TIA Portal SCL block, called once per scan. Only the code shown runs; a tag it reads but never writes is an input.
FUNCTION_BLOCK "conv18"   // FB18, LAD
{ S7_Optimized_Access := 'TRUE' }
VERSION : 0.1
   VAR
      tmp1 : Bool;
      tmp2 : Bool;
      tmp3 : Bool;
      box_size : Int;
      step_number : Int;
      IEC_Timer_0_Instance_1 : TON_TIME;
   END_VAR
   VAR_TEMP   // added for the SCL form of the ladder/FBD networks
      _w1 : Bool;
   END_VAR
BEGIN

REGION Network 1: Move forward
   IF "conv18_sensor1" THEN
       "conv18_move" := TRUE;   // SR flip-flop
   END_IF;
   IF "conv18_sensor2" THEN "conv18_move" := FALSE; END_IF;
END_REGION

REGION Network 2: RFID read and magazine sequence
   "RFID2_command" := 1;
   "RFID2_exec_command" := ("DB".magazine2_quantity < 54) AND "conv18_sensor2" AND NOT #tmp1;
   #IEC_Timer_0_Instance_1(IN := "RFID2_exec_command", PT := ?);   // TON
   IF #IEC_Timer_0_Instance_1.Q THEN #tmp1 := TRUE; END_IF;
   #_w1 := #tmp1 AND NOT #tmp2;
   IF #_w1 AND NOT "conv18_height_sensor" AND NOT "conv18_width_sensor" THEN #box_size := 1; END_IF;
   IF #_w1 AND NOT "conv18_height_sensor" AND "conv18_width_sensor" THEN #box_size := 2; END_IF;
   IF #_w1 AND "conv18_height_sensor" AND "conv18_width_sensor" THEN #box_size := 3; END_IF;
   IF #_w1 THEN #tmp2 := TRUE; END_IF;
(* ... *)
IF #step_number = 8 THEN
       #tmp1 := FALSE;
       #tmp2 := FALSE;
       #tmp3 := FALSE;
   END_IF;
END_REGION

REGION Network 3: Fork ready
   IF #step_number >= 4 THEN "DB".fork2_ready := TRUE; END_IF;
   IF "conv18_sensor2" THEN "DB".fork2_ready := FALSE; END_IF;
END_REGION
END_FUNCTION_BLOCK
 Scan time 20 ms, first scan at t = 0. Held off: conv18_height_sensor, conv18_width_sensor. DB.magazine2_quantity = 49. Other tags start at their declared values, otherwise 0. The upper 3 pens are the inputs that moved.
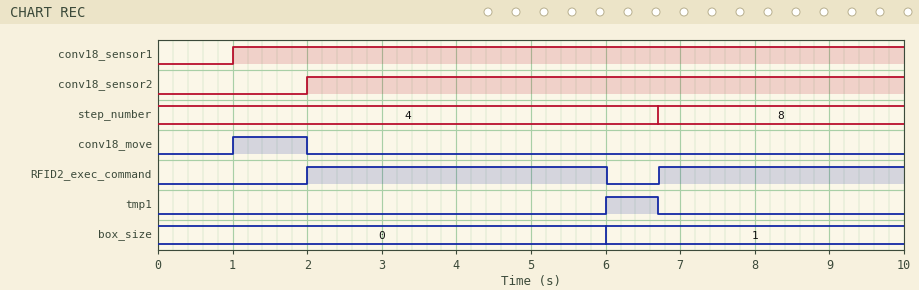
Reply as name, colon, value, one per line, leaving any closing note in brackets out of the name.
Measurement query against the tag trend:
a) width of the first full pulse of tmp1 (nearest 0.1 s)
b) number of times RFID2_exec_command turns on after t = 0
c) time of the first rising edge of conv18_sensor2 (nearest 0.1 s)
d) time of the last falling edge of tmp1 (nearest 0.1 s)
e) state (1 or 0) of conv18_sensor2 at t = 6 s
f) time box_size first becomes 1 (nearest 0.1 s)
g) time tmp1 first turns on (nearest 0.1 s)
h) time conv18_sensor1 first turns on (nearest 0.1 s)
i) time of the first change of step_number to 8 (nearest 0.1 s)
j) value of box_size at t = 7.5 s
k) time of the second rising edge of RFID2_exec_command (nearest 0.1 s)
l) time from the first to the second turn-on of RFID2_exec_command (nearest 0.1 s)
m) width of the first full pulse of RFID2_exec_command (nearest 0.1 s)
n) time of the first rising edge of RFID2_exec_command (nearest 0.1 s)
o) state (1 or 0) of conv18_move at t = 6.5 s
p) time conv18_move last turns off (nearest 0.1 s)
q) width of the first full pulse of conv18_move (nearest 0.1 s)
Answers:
width of the first full pulse of tmp1: 0.7 s
number of times RFID2_exec_command turns on after t = 0: 2
time of the first rising edge of conv18_sensor2: 2.0 s
time of the last falling edge of tmp1: 6.7 s
state (1 or 0) of conv18_sensor2 at t = 6 s: 1
time box_size first becomes 1: 6.0 s
time tmp1 first turns on: 6.0 s
time conv18_sensor1 first turns on: 1.0 s
time of the first change of step_number to 8: 6.7 s
value of box_size at t = 7.5 s: 1
time of the second rising edge of RFID2_exec_command: 6.7 s
time from the first to the second turn-on of RFID2_exec_command: 4.7 s
width of the first full pulse of RFID2_exec_command: 4.0 s
time of the first rising edge of RFID2_exec_command: 2.0 s
state (1 or 0) of conv18_move at t = 6.5 s: 0
time conv18_move last turns off: 2.0 s
width of the first full pulse of conv18_move: 1.0 s
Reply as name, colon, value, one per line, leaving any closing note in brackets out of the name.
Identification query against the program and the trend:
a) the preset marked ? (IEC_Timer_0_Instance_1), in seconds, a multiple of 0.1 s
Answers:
the preset marked ? (IEC_Timer_0_Instance_1), in seconds, a multiple of 0.1 s: 4.0 s
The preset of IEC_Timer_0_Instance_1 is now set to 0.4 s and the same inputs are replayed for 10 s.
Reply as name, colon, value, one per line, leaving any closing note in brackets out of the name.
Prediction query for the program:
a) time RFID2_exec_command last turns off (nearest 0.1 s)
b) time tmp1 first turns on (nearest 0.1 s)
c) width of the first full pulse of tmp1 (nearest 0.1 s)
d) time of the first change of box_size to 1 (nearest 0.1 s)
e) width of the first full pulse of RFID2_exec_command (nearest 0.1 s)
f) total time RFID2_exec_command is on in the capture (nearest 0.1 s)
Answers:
time RFID2_exec_command last turns off: 2.4 s
time tmp1 first turns on: 2.4 s
width of the first full pulse of tmp1: 4.3 s
time of the first change of box_size to 1: 2.4 s
width of the first full pulse of RFID2_exec_command: 0.4 s
total time RFID2_exec_command is on in the capture: 3.7 s
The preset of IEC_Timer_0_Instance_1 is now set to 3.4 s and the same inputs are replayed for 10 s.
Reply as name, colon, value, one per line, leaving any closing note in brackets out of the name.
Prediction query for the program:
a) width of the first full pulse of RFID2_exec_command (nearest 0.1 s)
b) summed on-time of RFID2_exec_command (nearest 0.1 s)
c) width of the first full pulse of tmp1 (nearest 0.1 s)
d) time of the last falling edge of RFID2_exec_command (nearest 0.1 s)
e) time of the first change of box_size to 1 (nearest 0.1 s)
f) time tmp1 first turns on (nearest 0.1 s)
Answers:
width of the first full pulse of RFID2_exec_command: 3.4 s
summed on-time of RFID2_exec_command: 6.7 s
width of the first full pulse of tmp1: 1.3 s
time of the last falling edge of RFID2_exec_command: 5.4 s
time of the first change of box_size to 1: 5.4 s
time tmp1 first turns on: 5.4 s
